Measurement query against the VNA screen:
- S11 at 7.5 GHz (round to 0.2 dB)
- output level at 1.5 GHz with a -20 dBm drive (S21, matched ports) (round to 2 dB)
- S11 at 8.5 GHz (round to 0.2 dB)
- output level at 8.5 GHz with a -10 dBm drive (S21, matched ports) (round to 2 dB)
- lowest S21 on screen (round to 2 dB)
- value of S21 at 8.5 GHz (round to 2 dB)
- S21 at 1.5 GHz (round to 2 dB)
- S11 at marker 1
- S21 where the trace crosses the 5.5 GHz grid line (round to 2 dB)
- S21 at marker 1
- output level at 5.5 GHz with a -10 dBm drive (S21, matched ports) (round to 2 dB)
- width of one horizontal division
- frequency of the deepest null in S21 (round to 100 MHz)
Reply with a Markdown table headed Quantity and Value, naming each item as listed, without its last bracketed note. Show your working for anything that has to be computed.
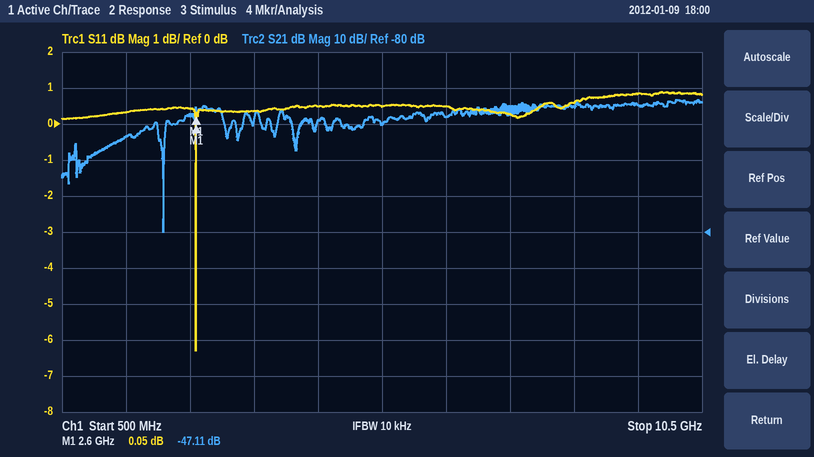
| Quantity | Value |
|---|---|
| S11 at 7.5 GHz | 0.2 dB |
| output level at 1.5 GHz with a -20 dBm drive (S21, matched ports) | -20 dBm + (-54 dB) = -74 dBm |
| S11 at 8.5 GHz | 0.6 dB |
| output level at 8.5 GHz with a -10 dBm drive (S21, matched ports) | -10 dBm + (-46 dB) = -56 dBm |
| lowest S21 on screen | -80 dB |
| value of S21 at 8.5 GHz | -46 dB |
| S21 at 1.5 GHz | -54 dB |
| S11 at marker 1 | 0.05 dB |
| S21 where the trace crosses the 5.5 GHz grid line | -50 dB |
| S21 at marker 1 | -47.11 dB |
| output level at 5.5 GHz with a -10 dBm drive (S21, matched ports) | -10 dBm + (-50 dB) = -60 dBm |
| width of one horizontal division | 1 GHz |
| frequency of the deepest null in S21 | 2.1 GHz |
